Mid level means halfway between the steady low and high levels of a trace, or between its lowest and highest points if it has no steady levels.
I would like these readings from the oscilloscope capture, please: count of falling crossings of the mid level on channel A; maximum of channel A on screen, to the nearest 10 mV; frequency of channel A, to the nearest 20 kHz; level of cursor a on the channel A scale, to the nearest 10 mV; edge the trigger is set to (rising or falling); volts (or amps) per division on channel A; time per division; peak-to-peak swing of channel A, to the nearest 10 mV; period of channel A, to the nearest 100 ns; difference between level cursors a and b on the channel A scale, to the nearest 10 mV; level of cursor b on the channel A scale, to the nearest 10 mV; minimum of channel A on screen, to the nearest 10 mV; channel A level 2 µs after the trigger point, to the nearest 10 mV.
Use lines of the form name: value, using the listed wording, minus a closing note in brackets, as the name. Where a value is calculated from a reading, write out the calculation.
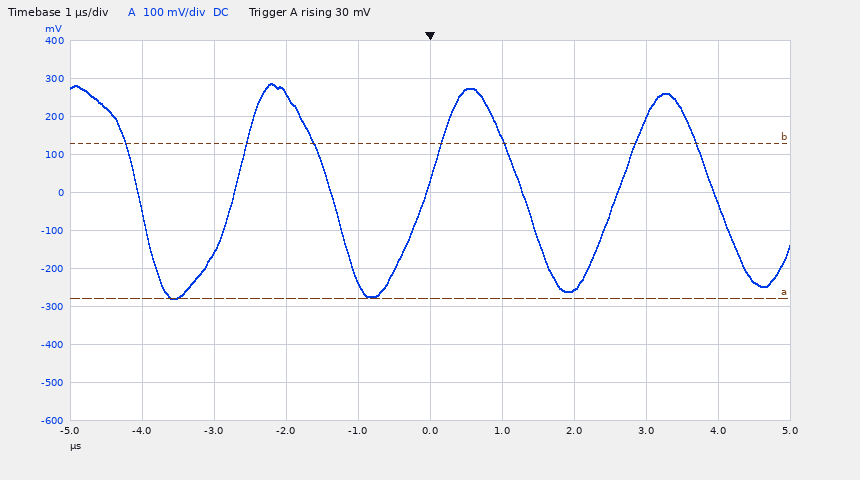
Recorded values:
count of falling crossings of the mid level on channel A: 4
maximum of channel A on screen, to the nearest 10 mV: 290 mV
frequency of channel A, to the nearest 20 kHz: 1 / 2.7 µs ≈ 370 kHz, so 380 kHz to the nearest 20 kHz
level of cursor a on the channel A scale, to the nearest 10 mV: -280 mV
edge the trigger is set to: rising
volts (or amps) per division on channel A: 100 mV
time per division: 1 µs
peak-to-peak swing of channel A, to the nearest 10 mV: 290 mV − (-280 mV) = 570 mV
period of channel A, to the nearest 100 ns: 2.7 µs
difference between level cursors a and b on the channel A scale, to the nearest 10 mV: 410 mV
level of cursor b on the channel A scale, to the nearest 10 mV: 130 mV
minimum of channel A on screen, to the nearest 10 mV: -280 mV
channel A level 2 µs after the trigger point, to the nearest 10 mV: -260 mV
